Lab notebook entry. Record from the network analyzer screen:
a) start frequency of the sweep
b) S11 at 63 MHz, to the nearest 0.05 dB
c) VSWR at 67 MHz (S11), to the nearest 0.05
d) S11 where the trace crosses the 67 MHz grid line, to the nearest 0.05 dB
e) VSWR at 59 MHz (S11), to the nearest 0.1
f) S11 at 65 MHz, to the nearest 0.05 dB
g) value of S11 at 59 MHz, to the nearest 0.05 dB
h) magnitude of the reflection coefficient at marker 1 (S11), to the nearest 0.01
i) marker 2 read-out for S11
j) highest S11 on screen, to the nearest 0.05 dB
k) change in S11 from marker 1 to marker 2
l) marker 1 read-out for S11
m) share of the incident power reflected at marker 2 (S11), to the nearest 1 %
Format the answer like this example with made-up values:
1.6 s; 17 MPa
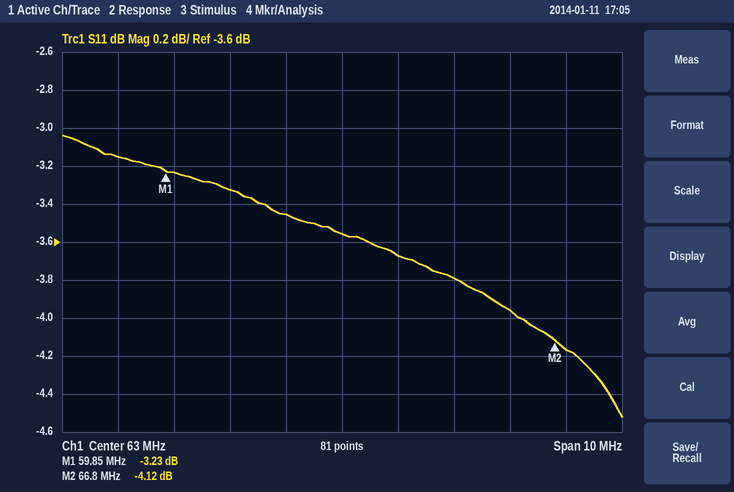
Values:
58 MHz; -3.55 dB; 4.25; -4.15 dB; 5.6; -3.80 dB; -3.15 dB; 0.69; -4.12 dB; -3.05 dB; -0.89 dB; -3.23 dB; 39 %
